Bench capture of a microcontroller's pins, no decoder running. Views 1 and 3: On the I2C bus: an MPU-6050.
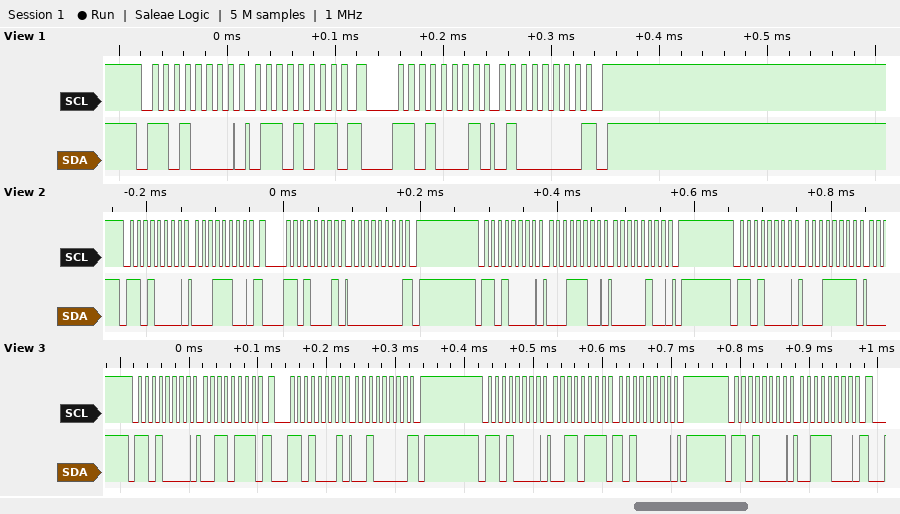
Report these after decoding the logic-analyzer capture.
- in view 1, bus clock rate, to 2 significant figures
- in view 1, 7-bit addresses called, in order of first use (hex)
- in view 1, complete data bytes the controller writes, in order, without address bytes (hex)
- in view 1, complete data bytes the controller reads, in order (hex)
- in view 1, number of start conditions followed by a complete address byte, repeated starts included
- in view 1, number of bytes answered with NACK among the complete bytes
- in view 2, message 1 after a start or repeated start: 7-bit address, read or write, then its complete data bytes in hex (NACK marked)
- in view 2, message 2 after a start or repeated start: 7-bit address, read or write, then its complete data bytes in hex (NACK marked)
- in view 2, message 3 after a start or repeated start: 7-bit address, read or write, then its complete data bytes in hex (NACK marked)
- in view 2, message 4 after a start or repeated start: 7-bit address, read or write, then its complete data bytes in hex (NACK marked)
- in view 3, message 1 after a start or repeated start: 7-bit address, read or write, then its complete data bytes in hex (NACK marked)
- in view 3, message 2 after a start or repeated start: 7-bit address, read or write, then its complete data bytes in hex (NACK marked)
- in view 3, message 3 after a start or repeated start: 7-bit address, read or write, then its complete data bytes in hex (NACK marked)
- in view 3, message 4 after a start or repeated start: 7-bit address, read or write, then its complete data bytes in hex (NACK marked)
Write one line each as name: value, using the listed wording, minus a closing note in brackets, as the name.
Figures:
in view 1, bus clock rate, to 2 significant figures: 100 kHz
in view 1, 7-bit addresses called, in order of first use: 0x68
in view 1, complete data bytes the controller writes, in order, without address bytes: 6B
in view 1, complete data bytes the controller reads, in order: 40
in view 1, number of start conditions followed by a complete address byte, repeated starts included: 2
in view 1, number of bytes answered with NACK among the complete bytes: 1
in view 2, message 1 after a start or repeated start: 7-bit address, read or write, then its complete data bytes in hex: 0x68 write: 1C
in view 2, message 2 after a start or repeated start: 7-bit address, read or write, then its complete data bytes in hex: 0x68 read: 00 NACK
in view 2, message 3 after a start or repeated start: 7-bit address, read or write, then its complete data bytes in hex: 0x68 write: 1C 04
in view 2, message 4 after a start or repeated start: 7-bit address, read or write, then its complete data bytes in hex: 0x68 write: 1F
in view 3, message 1 after a start or repeated start: 7-bit address, read or write, then its complete data bytes in hex: 0x68 write: 37
in view 3, message 2 after a start or repeated start: 7-bit address, read or write, then its complete data bytes in hex: 0x68 read: 20 NACK
in view 3, message 3 after a start or repeated start: 7-bit address, read or write, then its complete data bytes in hex: 0x68 write: 37 A0
in view 3, message 4 after a start or repeated start: 7-bit address, read or write, then its complete data bytes in hex: 0x68 write: 38
